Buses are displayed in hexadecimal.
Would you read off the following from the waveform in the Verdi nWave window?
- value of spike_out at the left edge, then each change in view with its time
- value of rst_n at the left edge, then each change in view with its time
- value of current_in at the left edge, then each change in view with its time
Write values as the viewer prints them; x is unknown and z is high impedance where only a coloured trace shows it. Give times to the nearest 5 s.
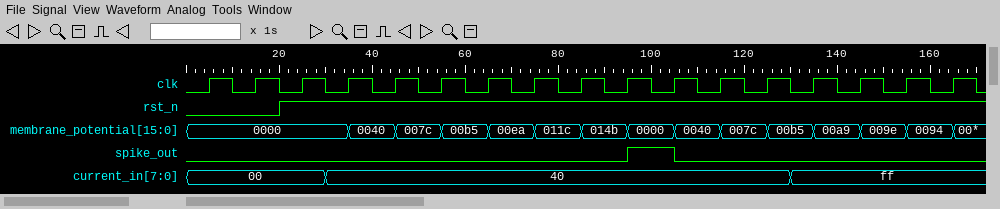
0, 1 at 95 s, 0 at 105 s
0, 1 at 20 s
00, 40 at 30 s, ff at 130 s
